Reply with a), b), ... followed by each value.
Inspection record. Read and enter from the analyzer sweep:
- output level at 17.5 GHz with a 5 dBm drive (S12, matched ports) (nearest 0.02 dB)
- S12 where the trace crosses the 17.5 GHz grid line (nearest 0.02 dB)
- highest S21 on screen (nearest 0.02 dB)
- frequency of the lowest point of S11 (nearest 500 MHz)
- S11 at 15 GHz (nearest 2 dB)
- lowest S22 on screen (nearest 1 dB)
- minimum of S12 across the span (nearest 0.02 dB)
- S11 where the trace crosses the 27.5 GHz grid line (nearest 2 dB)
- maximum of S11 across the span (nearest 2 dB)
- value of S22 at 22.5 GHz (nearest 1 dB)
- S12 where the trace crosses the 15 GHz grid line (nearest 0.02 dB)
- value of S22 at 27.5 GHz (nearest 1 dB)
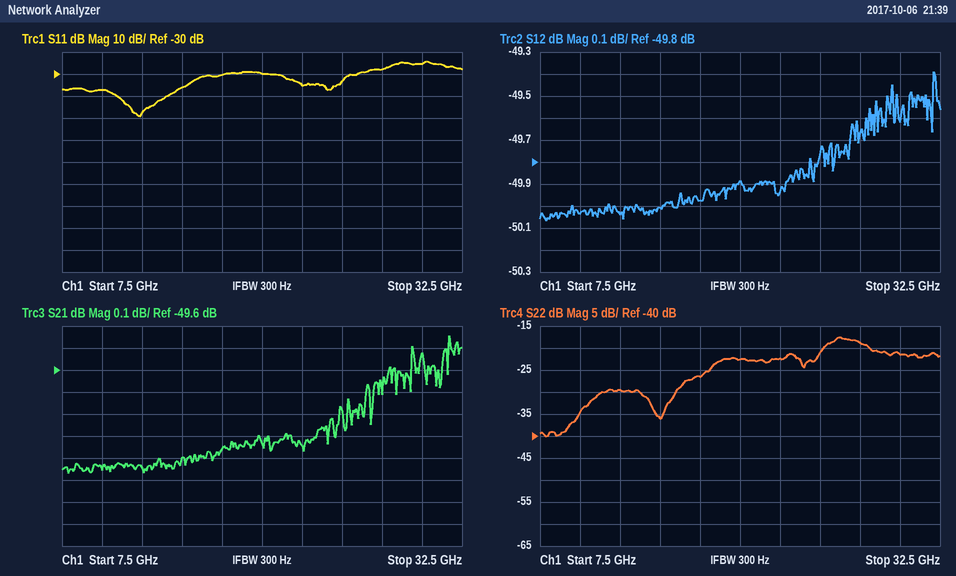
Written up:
a) -44.98 dBm
b) -49.98 dB
c) -49.44 dB
d) 12.5 GHz
e) -36 dB
f) -40 dB
g) -50.06 dB
h) -28 dB
i) -24 dB
j) -22 dB
k) -50.00 dB
l) -19 dB
